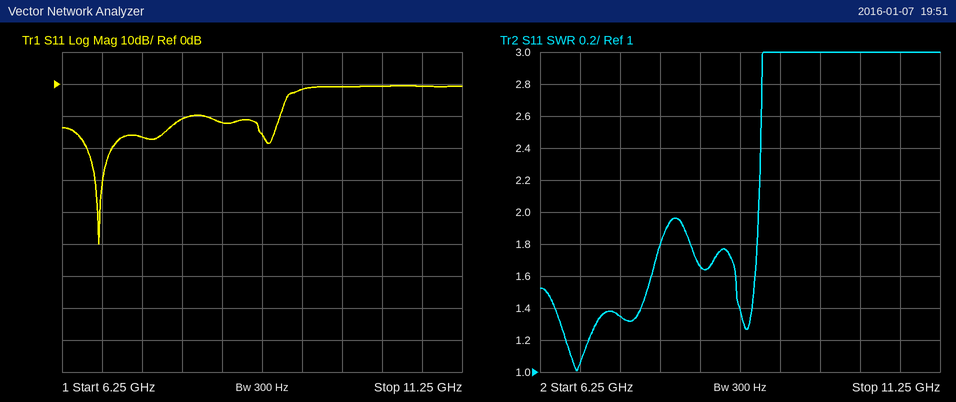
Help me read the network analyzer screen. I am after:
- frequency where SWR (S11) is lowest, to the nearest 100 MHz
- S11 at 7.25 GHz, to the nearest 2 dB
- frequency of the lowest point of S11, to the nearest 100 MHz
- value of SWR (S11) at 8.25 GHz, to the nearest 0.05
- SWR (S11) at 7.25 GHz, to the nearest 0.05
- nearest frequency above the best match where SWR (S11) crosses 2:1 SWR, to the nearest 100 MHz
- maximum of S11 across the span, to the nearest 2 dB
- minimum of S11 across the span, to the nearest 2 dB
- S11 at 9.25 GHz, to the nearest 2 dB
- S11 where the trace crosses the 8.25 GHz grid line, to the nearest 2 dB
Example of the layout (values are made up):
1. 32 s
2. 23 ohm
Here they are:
1. 6.7 GHz
2. -16 dB
3. 6.7 GHz
4. 1.65
5. 1.35
6. 9.0 GHz
7. 0 dB
8. -50 dB
9. -2 dB
10. -12 dB
